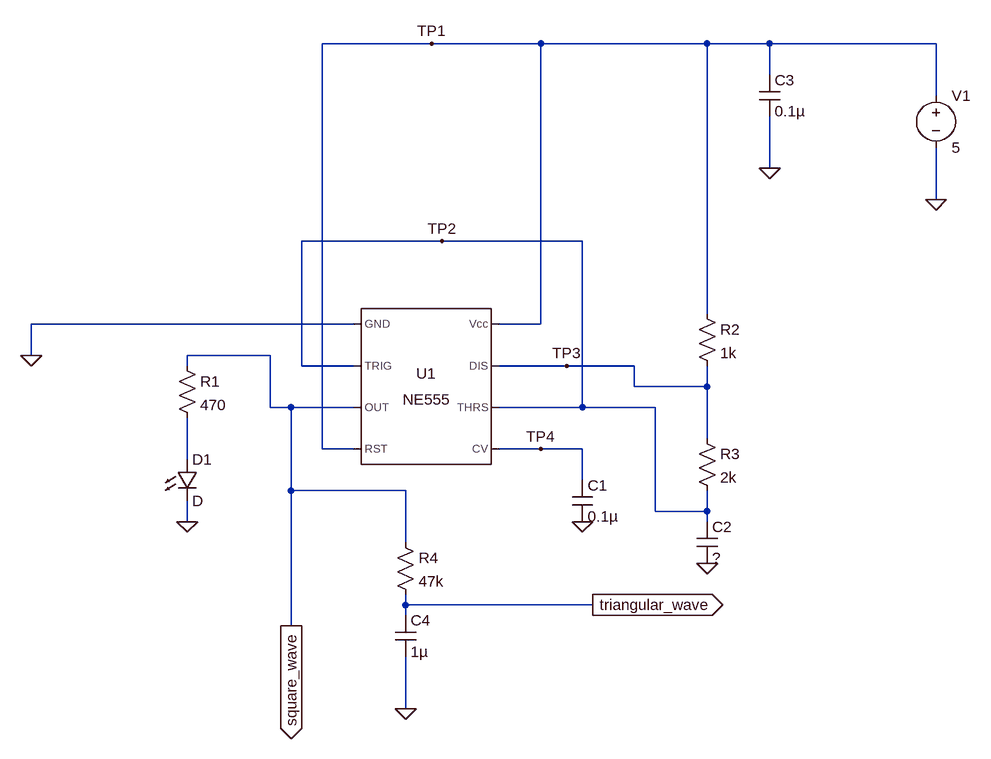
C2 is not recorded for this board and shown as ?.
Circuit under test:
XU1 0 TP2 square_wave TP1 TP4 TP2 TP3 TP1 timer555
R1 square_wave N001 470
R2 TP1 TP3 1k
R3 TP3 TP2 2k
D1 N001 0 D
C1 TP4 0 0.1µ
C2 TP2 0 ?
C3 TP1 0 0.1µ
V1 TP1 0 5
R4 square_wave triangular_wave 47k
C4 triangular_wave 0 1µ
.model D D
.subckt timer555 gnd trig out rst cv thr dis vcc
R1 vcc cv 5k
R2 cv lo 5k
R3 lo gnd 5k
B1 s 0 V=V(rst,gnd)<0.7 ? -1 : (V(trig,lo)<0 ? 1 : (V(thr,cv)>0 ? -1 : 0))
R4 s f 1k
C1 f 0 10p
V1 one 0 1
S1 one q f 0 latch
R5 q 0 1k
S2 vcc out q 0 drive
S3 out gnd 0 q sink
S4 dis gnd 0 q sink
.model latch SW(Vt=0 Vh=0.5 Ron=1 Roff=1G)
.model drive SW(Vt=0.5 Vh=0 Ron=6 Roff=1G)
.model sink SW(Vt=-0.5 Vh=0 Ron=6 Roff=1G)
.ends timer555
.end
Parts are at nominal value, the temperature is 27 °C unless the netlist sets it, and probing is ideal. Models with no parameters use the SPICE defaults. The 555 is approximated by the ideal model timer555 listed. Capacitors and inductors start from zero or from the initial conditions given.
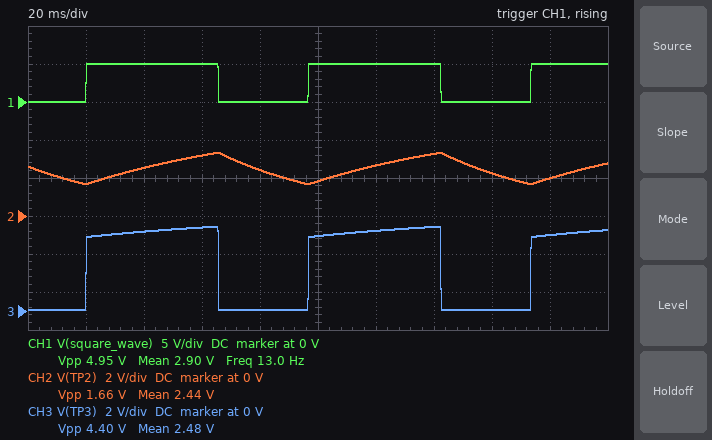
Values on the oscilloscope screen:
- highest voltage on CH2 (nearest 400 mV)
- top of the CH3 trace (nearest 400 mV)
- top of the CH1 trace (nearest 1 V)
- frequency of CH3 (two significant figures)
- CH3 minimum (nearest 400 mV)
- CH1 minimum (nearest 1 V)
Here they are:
3.2 V
4.4 V
5 V
13 Hz
0 V
0 V
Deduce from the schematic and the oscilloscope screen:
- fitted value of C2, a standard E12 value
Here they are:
22 µF
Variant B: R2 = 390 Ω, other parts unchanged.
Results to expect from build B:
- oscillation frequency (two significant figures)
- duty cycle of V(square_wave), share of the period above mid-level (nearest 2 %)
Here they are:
15 Hz
54 %
